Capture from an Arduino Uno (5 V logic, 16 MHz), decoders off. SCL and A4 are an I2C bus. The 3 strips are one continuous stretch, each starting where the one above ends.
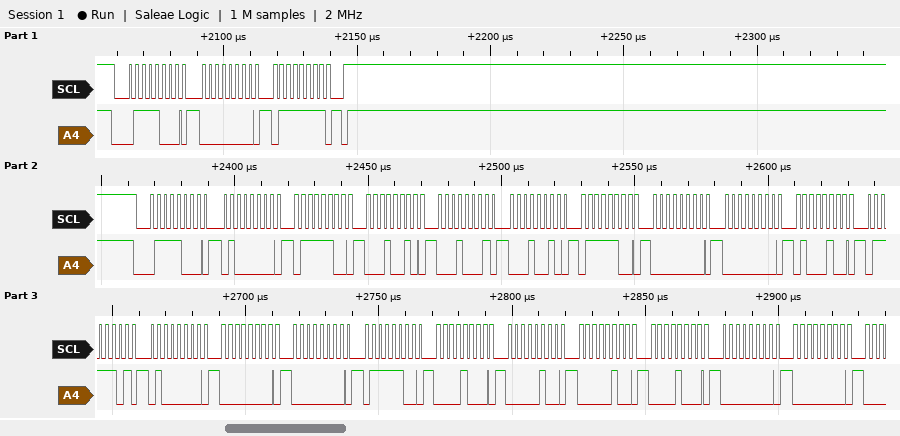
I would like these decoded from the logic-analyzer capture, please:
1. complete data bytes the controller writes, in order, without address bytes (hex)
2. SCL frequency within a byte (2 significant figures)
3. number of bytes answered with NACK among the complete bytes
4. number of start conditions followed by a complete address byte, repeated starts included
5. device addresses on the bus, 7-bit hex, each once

00 7F 40 7C 12 11 12 7C 00 00 44 7D 40 00 00 7C 08 04 04 08 00 00
400 kHz
0
2
0x3C
